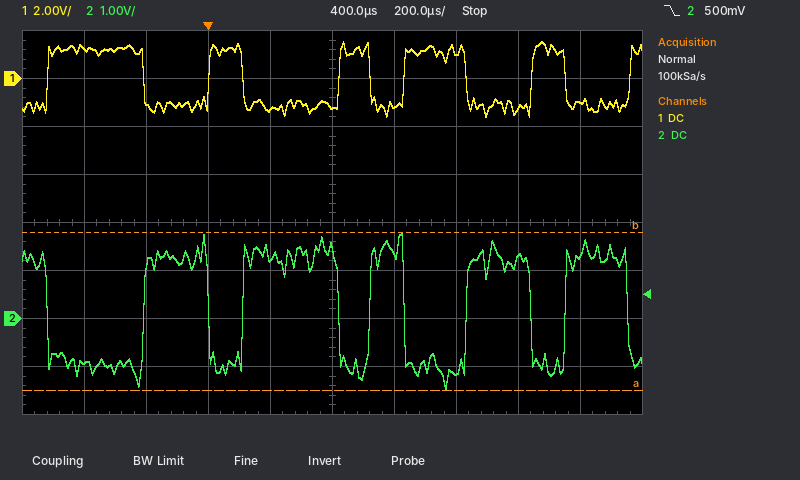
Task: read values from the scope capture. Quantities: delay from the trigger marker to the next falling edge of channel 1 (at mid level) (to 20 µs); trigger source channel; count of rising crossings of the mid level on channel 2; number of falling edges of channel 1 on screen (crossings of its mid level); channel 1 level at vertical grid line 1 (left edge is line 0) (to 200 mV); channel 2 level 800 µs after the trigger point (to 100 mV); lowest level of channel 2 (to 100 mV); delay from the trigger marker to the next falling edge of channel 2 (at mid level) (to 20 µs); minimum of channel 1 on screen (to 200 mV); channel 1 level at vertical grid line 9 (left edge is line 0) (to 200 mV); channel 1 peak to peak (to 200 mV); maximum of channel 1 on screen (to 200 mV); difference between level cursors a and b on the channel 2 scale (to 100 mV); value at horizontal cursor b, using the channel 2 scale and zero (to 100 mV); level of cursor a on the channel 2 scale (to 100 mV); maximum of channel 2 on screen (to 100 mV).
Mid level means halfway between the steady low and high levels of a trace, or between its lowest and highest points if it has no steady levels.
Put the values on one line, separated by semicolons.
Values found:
120 µs; channel 2; 5; 5; 1.2 V; -1.1 V; -1.5 V; 420 µs; -1.6 V; -1.0 V; 3.2 V; 1.6 V; 3.3 V; 1.8 V; -1.5 V; 1.8 V
